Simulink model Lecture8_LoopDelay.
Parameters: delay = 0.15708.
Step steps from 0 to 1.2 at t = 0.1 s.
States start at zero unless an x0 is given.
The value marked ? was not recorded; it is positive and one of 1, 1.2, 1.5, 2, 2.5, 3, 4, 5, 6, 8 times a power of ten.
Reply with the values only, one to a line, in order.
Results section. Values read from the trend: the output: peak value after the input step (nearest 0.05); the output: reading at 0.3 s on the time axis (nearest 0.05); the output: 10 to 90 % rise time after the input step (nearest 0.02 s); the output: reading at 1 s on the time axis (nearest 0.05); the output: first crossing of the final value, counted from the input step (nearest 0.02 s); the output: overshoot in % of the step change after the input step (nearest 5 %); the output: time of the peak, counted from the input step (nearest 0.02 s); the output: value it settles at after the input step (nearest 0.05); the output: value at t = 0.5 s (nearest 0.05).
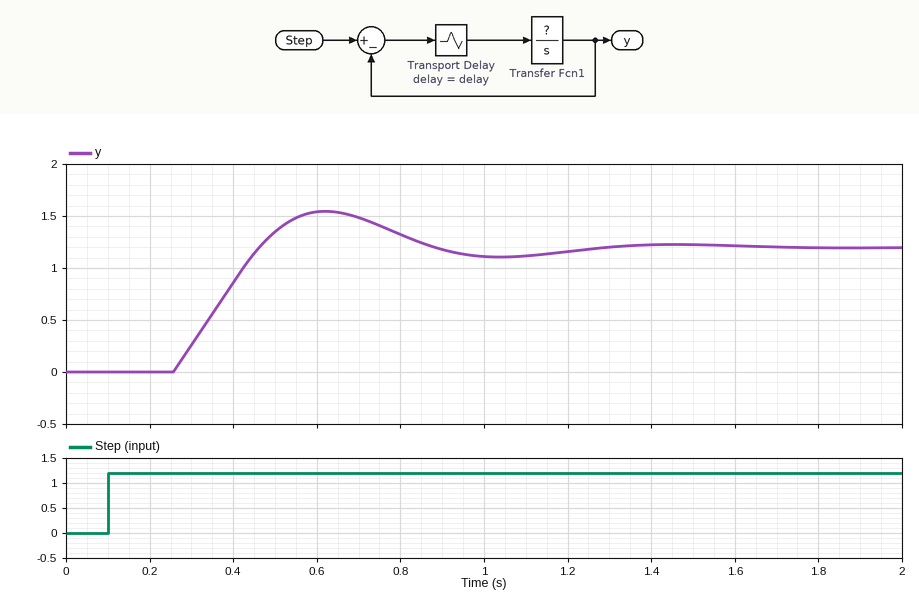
1.55
0.25
0.16 s
1.10
0.36 s
30 %
0.52 s
1.20
1.35
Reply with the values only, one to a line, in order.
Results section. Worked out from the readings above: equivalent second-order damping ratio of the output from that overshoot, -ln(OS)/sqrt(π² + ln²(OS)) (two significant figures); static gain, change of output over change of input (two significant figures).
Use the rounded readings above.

0.36
1.0
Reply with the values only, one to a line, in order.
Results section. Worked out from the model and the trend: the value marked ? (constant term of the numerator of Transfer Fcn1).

5
